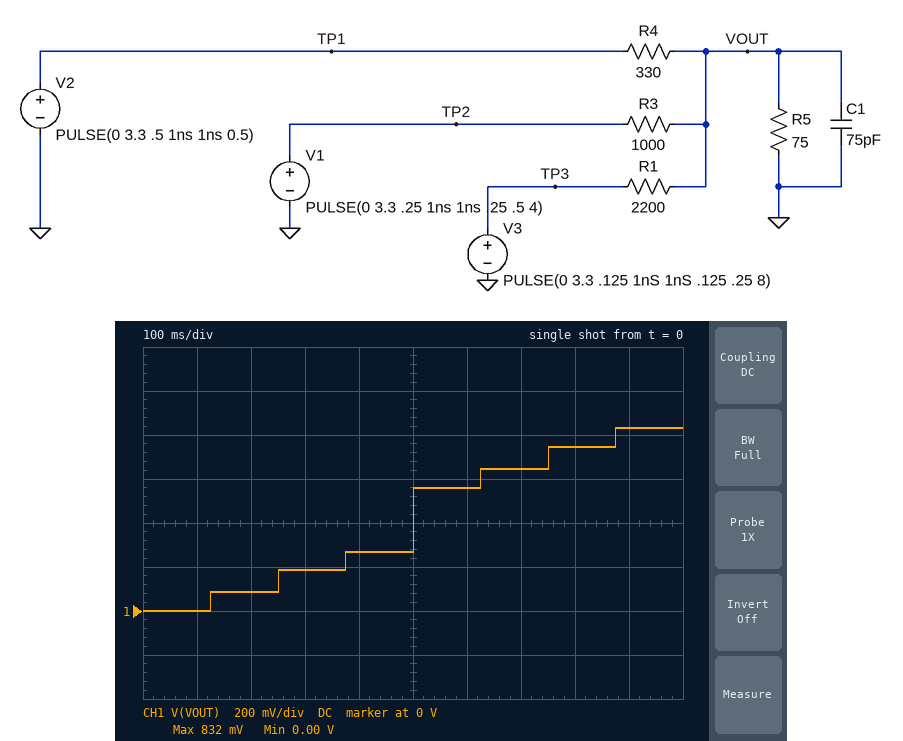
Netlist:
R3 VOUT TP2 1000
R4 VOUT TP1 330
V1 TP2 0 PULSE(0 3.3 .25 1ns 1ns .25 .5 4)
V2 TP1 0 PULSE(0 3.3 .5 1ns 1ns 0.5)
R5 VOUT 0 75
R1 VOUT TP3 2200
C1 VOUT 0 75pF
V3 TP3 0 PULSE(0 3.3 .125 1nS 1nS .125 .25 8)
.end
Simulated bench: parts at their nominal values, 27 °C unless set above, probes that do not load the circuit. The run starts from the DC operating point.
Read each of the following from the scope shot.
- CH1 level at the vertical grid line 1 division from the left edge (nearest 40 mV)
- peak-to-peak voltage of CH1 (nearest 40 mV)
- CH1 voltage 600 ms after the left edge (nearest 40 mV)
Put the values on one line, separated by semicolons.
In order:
0 V; 840 mV; 560 mV
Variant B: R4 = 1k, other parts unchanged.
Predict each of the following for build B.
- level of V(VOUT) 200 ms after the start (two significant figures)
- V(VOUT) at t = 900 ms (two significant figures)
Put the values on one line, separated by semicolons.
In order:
95 mV; 510 mV
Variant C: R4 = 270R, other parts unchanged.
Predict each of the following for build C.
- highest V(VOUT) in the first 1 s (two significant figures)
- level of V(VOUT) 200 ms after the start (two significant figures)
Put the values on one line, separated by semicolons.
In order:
920 mV; 81 mV
